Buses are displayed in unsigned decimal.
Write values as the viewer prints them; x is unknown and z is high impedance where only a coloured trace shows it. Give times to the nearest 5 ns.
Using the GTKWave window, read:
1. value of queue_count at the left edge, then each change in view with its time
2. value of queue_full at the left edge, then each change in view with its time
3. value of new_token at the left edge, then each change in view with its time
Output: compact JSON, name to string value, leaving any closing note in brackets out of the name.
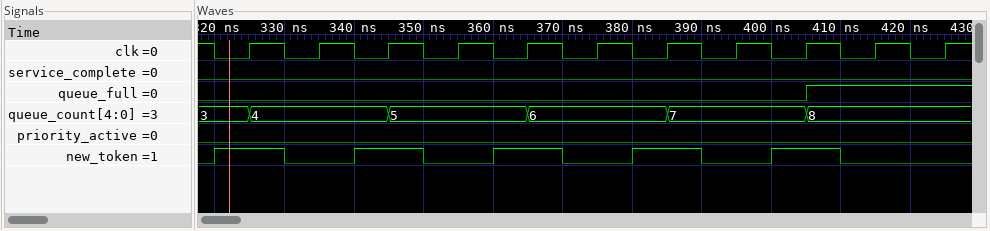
{"value of queue_count at the left edge, then each change in view with its time": "3, 4 at 325 ns, 5 at 345 ns, 6 at 365 ns, 7 at 385 ns, 8 at 405 ns", "value of queue_full at the left edge, then each change in view with its time": "0, 1 at 405 ns", "value of new_token at the left edge, then each change in view with its time": "0, 1 at 320 ns, 0 at 330 ns, 1 at 340 ns, 0 at 350 ns, 1 at 360 ns, 0 at 370 ns, 1 at 380 ns, 0 at 390 ns, 1 at 400 ns, 0 at 410 ns"}
